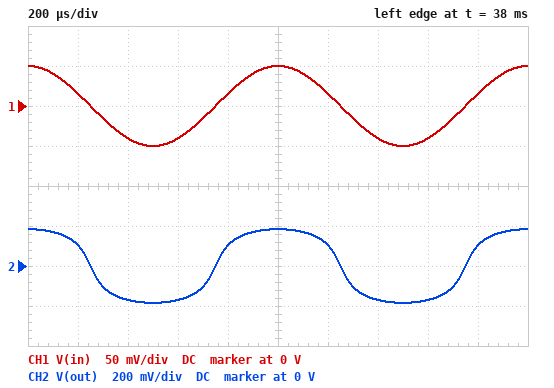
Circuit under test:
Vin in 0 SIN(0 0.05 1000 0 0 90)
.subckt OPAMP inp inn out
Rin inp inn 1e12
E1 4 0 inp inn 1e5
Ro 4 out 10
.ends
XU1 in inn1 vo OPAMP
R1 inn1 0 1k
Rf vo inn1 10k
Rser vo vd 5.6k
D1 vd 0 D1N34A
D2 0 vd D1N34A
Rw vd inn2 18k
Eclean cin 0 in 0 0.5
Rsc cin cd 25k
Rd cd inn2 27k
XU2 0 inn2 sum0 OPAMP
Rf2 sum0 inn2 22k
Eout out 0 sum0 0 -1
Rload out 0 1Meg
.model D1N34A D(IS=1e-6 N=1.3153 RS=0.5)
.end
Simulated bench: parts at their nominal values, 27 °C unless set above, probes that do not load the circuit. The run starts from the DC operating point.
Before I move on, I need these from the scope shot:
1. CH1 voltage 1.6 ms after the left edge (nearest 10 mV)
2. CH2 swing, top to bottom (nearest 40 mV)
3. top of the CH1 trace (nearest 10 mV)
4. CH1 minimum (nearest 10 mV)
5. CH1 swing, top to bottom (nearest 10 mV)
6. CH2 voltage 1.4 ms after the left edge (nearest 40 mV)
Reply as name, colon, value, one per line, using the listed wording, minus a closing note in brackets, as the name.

CH1 voltage 1.6 ms after the left edge: -40 mV
CH2 swing, top to bottom: 360 mV
top of the CH1 trace: 50 mV
CH1 minimum: -50 mV
CH1 swing, top to bottom: 100 mV
CH2 voltage 1.4 ms after the left edge: -160 mV
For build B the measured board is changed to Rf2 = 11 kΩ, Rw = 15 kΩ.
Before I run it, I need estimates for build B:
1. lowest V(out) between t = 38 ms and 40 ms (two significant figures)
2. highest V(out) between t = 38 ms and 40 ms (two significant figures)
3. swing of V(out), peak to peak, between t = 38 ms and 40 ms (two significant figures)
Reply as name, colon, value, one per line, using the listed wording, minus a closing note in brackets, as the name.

lowest V(out) between t = 38 ms and 40 ms: -110 mV
highest V(out) between t = 38 ms and 40 ms: 110 mV
swing of V(out), peak to peak, between t = 38 ms and 40 ms: 220 mV
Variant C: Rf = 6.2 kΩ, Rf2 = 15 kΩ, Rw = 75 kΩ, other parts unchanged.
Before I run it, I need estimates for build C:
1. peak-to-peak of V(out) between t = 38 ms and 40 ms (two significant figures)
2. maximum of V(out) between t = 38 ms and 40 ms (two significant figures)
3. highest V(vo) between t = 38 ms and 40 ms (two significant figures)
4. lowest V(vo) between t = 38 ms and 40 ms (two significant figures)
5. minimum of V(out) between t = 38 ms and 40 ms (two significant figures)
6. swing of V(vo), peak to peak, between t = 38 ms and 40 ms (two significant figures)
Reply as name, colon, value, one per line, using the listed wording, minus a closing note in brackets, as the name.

peak-to-peak of V(out) between t = 38 ms and 40 ms: 65 mV
maximum of V(out) between t = 38 ms and 40 ms: 32 mV
highest V(vo) between t = 38 ms and 40 ms: 360 mV
lowest V(vo) between t = 38 ms and 40 ms: -360 mV
minimum of V(out) between t = 38 ms and 40 ms: -32 mV
swing of V(vo), peak to peak, between t = 38 ms and 40 ms: 720 mV
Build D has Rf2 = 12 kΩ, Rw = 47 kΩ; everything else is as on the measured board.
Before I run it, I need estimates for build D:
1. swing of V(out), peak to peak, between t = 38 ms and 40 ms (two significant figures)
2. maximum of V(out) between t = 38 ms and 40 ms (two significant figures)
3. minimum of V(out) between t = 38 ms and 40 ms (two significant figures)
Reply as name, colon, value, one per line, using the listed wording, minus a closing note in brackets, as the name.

swing of V(out), peak to peak, between t = 38 ms and 40 ms: 85 mV
maximum of V(out) between t = 38 ms and 40 ms: 43 mV
minimum of V(out) between t = 38 ms and 40 ms: -43 mV
